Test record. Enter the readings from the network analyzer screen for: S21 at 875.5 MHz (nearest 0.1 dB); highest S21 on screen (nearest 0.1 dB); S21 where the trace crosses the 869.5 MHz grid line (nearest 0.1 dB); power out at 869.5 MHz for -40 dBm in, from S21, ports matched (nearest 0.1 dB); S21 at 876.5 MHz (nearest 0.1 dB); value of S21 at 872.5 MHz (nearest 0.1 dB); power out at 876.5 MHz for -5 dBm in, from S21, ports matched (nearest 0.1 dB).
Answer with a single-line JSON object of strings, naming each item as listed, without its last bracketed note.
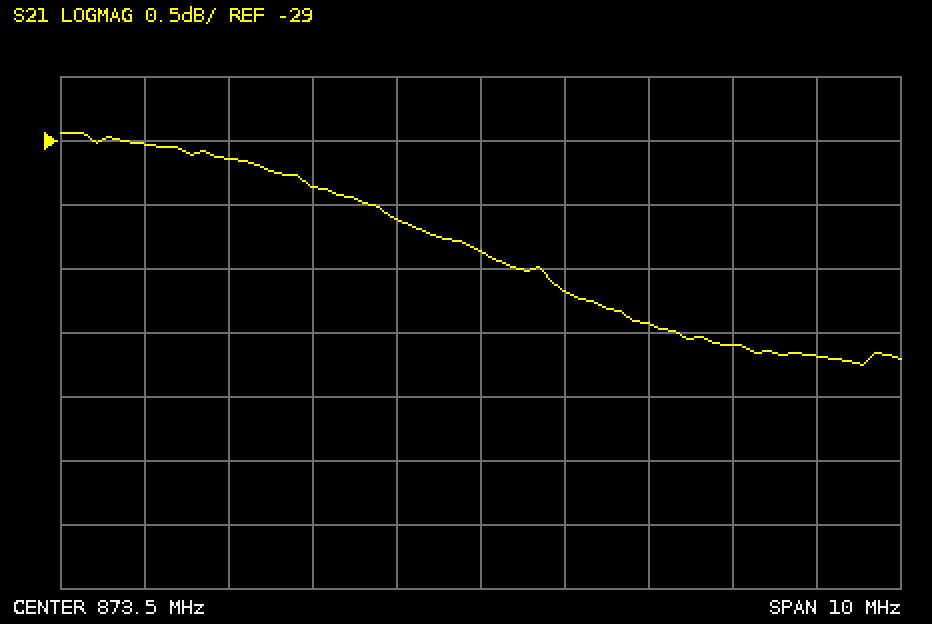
{"S21 at 875.5 MHz": "-30.4 dB", "highest S21 on screen": "-28.9 dB", "S21 where the trace crosses the 869.5 MHz grid line": "-29.0 dB", "power out at 869.5 MHz for -40 dBm in, from S21, ports matched": "-69.0 dBm", "S21 at 876.5 MHz": "-30.6 dB", "value of S21 at 872.5 MHz": "-29.6 dB", "power out at 876.5 MHz for -5 dBm in, from S21, ports matched": "-35.6 dBm"}
